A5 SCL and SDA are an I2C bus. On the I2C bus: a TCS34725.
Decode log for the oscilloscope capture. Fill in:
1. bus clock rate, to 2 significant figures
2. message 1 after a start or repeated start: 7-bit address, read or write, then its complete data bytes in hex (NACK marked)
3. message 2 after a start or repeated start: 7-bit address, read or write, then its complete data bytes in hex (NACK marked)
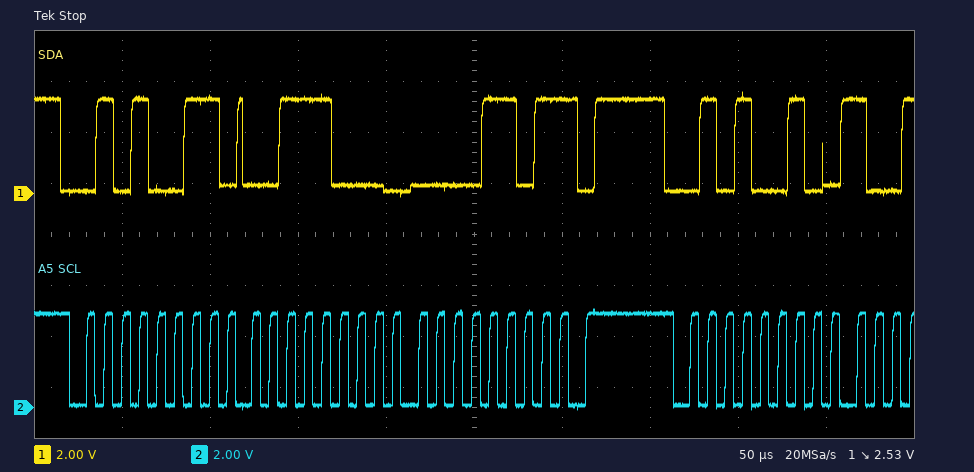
100 kHz
0x29 read: 38 0D NACK
0x29 write
